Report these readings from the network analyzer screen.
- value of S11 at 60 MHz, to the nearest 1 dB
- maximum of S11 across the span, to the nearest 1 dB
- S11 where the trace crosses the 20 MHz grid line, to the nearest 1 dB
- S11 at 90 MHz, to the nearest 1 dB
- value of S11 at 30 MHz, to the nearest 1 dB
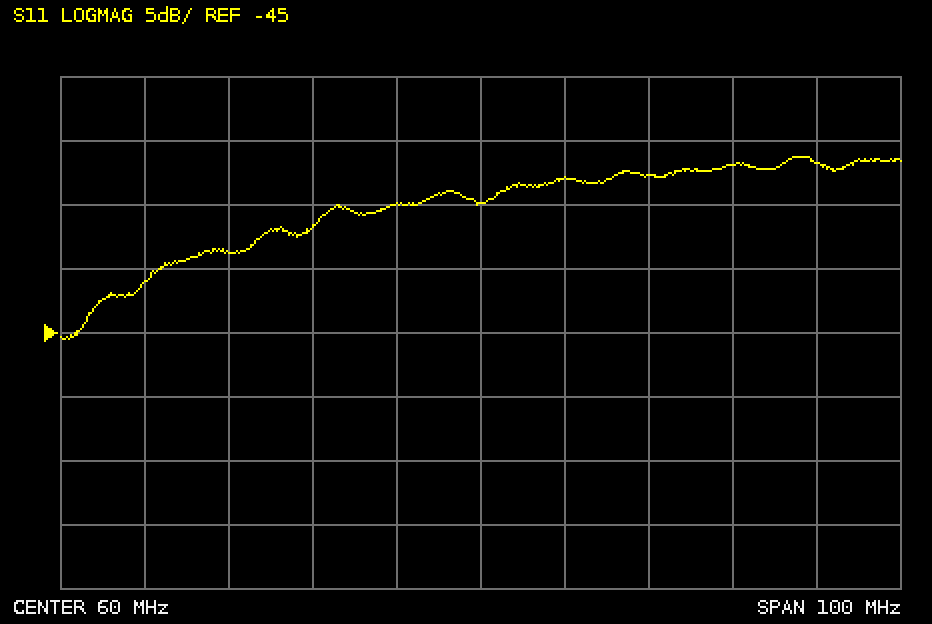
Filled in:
-35 dB
-31 dB
-41 dB
-32 dB
-39 dB
